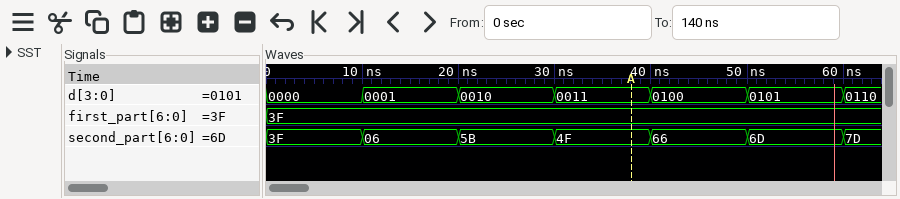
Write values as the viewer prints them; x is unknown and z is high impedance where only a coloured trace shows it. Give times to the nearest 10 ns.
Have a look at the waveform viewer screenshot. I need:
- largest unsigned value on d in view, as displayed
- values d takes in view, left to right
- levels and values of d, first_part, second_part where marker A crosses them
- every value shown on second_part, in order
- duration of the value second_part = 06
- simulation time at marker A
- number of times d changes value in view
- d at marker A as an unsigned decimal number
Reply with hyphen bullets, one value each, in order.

- 0110
- 0000, 0001, 0010, 0011, 0100, 0101, 0110
- d=0011, first_part=3F, second_part=4F
- 3F, 06, 5B, 4F, 66, 6D, 7D
- 10 ns
- 40 ns
- 6
- 3
